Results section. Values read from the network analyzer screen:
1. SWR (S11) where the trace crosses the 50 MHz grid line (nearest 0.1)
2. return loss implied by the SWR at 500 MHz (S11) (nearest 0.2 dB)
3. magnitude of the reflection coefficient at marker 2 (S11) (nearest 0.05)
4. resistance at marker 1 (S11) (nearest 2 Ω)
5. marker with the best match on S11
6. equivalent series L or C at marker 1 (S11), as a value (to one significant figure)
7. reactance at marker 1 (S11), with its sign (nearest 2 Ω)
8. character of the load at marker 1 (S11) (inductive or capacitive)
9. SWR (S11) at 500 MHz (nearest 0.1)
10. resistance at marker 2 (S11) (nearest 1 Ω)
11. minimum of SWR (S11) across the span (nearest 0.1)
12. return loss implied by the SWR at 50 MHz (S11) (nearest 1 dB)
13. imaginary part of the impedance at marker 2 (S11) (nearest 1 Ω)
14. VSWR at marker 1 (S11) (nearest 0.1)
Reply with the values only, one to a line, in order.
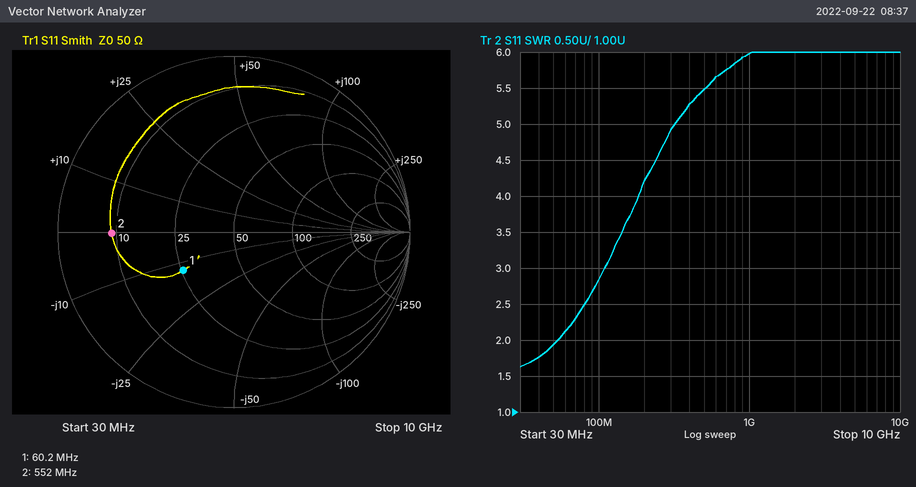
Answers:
1.9
3.2 dB
0.70
26 Ω
marker 1
200 pF
-12 Ω
capacitive
5.5
9 Ω
1.6
10 dB
0 Ω
2.1
